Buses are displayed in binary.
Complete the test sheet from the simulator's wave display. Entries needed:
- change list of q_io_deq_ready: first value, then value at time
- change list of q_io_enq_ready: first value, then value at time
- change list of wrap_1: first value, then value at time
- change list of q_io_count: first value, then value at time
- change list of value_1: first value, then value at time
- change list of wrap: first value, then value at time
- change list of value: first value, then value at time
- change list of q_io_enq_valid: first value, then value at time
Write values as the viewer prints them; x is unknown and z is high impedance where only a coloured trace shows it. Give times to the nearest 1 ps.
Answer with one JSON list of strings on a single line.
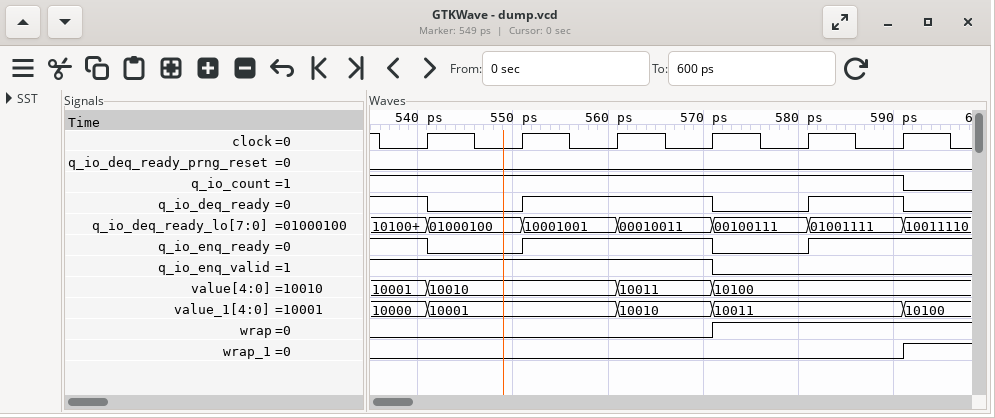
["1, 0 at 541 ps, 1 at 551 ps, 0 at 571 ps, 1 at 581 ps, 0 at 591 ps", "1, 0 at 541 ps, 1 at 551 ps, 0 at 571 ps, 1 at 581 ps", "0, 1 at 591 ps", "1, 0 at 591 ps", "10000, 10001 at 541 ps, 10010 at 561 ps, 10011 at 571 ps, 10100 at 591 ps", "0, 1 at 571 ps", "10001, 10010 at 541 ps, 10011 at 561 ps, 10100 at 571 ps", "1, 0 at 571 ps"]
